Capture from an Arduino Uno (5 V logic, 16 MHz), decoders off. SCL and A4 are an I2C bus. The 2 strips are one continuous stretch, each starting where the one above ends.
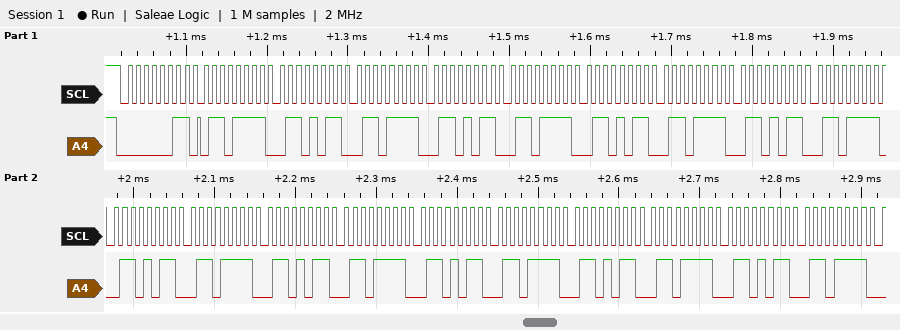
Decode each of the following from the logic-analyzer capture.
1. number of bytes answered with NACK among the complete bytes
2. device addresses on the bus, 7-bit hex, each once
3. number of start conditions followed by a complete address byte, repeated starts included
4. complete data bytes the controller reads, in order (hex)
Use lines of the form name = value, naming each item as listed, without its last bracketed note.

number of bytes answered with NACK among the complete bytes = 0
device addresses on the bus, 7-bit hex, each once = 0x01
number of start conditions followed by a complete address byte, repeated starts included = 1
complete data bytes the controller reads, in order = 6F 6B 6F 6B 6F 6B 6F 6B 6F 6B 6F 6B 6F 6B 6F 6B 6F 6B 6F
